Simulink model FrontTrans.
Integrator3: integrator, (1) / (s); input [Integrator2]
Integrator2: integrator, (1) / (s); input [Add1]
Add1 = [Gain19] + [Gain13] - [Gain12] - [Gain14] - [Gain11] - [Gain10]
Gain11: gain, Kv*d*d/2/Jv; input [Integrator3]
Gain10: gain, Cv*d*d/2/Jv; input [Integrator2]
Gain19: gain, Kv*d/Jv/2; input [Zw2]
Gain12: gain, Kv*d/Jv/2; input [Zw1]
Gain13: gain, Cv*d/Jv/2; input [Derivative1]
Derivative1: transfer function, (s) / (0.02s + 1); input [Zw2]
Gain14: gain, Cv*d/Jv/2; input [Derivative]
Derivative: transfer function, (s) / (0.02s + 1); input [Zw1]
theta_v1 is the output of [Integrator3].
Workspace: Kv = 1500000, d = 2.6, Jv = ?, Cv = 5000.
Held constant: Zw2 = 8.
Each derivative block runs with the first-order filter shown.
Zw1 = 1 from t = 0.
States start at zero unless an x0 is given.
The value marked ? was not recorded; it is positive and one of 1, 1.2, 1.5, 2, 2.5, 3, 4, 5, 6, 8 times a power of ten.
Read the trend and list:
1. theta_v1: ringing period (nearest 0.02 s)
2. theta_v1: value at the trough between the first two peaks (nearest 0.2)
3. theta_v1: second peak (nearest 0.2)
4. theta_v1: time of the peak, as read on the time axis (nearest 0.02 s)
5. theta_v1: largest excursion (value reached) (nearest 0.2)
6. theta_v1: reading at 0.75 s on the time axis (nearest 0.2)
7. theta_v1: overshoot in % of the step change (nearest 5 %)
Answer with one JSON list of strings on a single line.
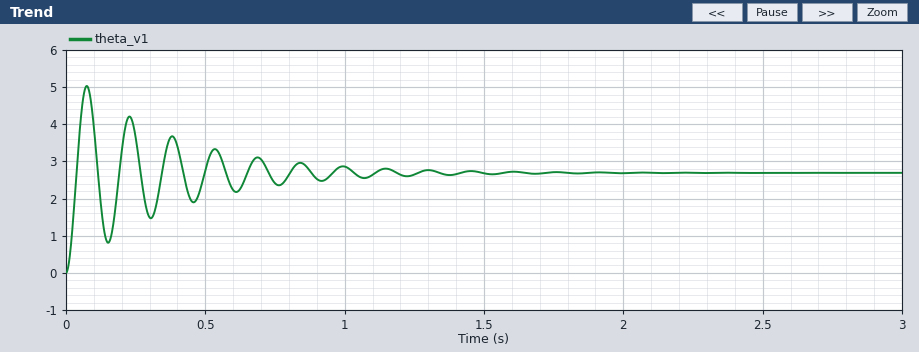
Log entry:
["0.16 s", "0.8", "4.2", "0.08 s", "5.0", "2.4", "85 %"]
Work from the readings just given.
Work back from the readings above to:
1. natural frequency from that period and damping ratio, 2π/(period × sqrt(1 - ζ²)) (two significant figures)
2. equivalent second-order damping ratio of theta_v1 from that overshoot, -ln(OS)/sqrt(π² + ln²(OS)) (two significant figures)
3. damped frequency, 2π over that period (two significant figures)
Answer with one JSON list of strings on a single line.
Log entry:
["39 rad/s", "0.052", "39 rad/s"]
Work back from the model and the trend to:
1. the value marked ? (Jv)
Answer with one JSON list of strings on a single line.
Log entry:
["3000"]
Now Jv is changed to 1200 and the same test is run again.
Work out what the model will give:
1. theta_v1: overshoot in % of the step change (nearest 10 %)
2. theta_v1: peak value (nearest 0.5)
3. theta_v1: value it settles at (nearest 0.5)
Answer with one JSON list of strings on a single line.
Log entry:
["80 %", "5.0", "2.5"]
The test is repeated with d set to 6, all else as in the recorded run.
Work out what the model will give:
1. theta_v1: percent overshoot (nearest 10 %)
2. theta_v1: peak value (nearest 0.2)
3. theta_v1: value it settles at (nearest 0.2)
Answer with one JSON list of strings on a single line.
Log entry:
["70 %", "2.0", "1.2"]
